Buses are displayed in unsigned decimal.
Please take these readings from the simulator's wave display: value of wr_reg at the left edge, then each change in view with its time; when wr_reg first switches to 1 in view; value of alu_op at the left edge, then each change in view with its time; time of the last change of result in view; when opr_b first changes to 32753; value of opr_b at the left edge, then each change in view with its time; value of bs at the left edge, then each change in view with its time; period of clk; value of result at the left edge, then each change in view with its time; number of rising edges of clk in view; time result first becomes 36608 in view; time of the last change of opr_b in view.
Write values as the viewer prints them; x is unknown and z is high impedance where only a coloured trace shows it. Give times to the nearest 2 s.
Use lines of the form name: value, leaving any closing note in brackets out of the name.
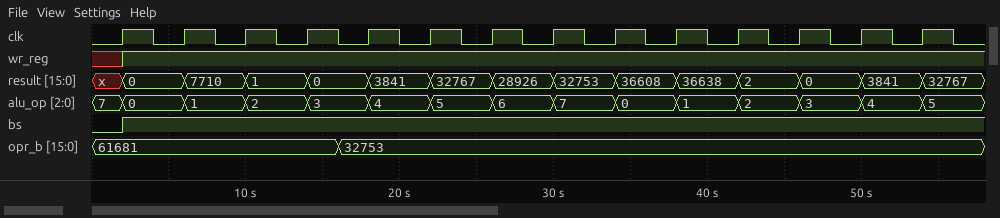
value of wr_reg at the left edge, then each change in view with its time: x, 1 at 2 s
when wr_reg first switches to 1 in view: 2 s
value of alu_op at the left edge, then each change in view with its time: 7, 0 at 2 s, 1 at 6 s, 2 at 10 s, 3 at 14 s, 4 at 18 s, 5 at 22 s, 6 at 26 s, 7 at 30 s, 0 at 34 s, 1 at 38 s, 2 at 42 s, 3 at 46 s, 4 at 50 s, 5 at 54 s
time of the last change of result in view: 54 s
when opr_b first changes to 32753: 16 s
value of opr_b at the left edge, then each change in view with its time: 61681, 32753 at 16 s
value of bs at the left edge, then each change in view with its time: 0, 1 at 2 s
period of clk: 4 s
value of result at the left edge, then each change in view with its time: x, 0 at 2 s, 7710 at 6 s, 1 at 10 s, 0 at 14 s, 3841 at 18 s, 32767 at 22 s, 28926 at 26 s, 32753 at 30 s, 36608 at 34 s, 36638 at 38 s, 2 at 42 s, 0 at 46 s, 3841 at 50 s, 32767 at 54 s
number of rising edges of clk in view: 14
time result first becomes 36608 in view: 34 s
time of the last change of opr_b in view: 16 s
